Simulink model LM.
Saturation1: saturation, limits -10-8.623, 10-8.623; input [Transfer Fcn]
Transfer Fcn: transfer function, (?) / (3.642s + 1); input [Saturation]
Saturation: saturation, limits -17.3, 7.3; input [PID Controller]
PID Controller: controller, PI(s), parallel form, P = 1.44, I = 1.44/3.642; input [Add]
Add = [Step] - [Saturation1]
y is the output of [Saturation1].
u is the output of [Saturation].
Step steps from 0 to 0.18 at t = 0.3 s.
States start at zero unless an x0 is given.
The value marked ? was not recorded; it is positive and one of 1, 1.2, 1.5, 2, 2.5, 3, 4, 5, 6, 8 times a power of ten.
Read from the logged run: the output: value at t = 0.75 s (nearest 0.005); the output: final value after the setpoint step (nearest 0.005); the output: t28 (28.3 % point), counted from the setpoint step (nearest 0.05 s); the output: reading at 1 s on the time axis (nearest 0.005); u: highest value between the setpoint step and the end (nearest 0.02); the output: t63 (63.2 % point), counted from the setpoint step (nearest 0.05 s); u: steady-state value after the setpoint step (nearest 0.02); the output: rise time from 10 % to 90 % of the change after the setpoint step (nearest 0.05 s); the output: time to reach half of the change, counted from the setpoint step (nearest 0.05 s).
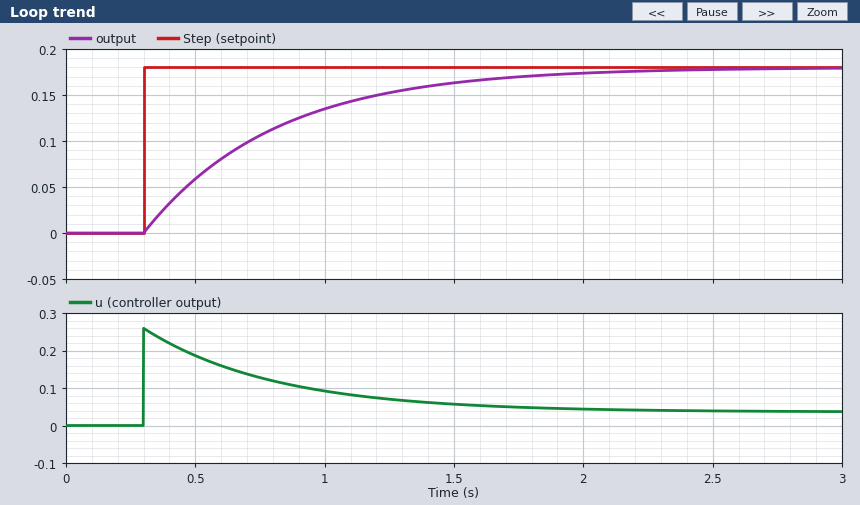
0.105
0.180
0.15 s
0.135
0.26
0.50 s
0.04
1.10 s
0.35 s
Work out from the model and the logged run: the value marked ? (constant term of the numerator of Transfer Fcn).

5
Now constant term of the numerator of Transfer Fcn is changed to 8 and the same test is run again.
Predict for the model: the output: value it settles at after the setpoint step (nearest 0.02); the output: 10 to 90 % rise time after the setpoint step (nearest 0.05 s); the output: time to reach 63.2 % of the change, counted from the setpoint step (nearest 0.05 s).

0.18
0.70 s
0.30 s
